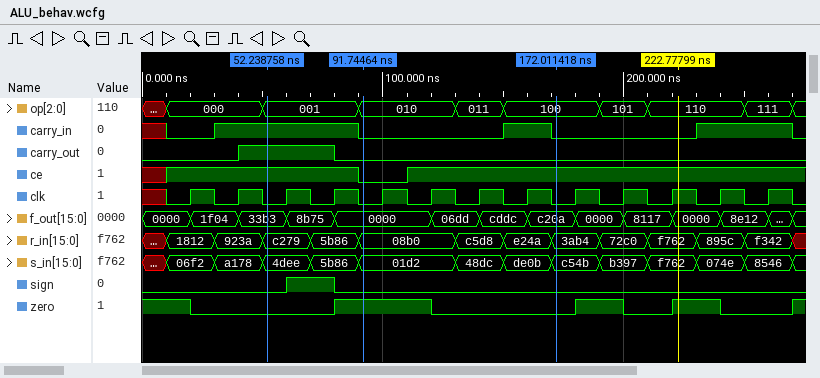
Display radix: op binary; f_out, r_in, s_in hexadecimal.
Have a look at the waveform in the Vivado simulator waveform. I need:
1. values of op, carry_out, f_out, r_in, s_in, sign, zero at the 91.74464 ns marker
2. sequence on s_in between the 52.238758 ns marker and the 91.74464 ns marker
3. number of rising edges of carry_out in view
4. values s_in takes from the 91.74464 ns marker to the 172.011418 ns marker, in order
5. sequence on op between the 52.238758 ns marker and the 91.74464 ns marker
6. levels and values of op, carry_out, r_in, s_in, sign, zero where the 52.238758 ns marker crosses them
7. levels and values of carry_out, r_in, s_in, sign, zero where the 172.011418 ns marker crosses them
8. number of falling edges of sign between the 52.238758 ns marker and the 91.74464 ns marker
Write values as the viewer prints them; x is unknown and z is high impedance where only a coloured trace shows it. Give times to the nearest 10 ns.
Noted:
op=010, carry_out=0, f_out=0000, r_in=08b0, s_in=01d2, sign=0, zero=1
4dee, 5b86, 01d2
1
01d2, 48dc, de0b, c54b
001, 010
op=001, carry_out=1, r_in=c279, s_in=4dee, sign=0, zero=0
carry_out=0, r_in=3ab4, s_in=c54b, sign=0, zero=0
1
